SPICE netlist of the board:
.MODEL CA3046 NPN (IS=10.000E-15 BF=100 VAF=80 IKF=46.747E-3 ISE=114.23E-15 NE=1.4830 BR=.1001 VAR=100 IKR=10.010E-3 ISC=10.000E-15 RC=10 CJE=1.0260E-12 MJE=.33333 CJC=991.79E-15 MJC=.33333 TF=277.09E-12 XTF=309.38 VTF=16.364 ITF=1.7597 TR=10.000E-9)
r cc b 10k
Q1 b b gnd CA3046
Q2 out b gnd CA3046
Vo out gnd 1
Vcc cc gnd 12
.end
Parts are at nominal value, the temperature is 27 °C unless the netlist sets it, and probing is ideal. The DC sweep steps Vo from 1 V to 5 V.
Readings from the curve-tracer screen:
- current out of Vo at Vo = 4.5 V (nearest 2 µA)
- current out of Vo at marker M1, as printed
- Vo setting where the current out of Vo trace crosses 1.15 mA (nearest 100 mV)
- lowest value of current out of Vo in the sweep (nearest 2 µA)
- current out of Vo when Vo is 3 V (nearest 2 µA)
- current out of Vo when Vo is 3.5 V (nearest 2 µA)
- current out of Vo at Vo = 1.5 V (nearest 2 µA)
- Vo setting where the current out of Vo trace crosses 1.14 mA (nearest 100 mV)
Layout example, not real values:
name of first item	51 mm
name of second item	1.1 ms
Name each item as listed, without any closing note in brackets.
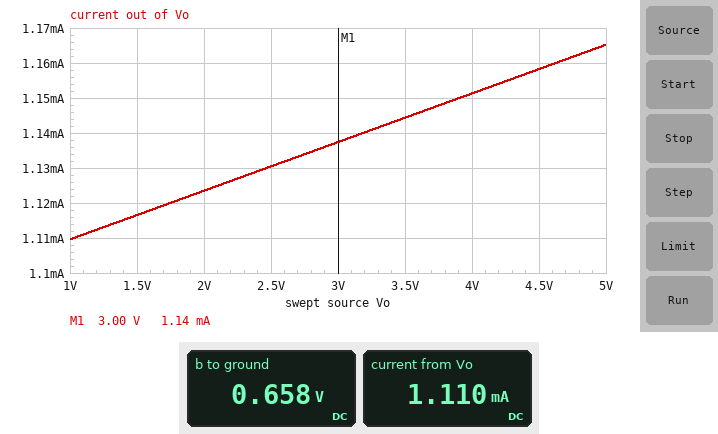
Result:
current out of Vo at Vo = 4.5 V	1.158 mA
current out of Vo at marker M1, as printed	1.14 mA
Vo setting where the current out of Vo trace crosses 1.15 mA	3.9 V
lowest value of current out of Vo in the sweep	1.110 mA
current out of Vo when Vo is 3 V	1.138 mA
current out of Vo when Vo is 3.5 V	1.144 mA
current out of Vo at Vo = 1.5 V	1.116 mA
Vo setting where the current out of Vo trace crosses 1.14 mA	3.2 V
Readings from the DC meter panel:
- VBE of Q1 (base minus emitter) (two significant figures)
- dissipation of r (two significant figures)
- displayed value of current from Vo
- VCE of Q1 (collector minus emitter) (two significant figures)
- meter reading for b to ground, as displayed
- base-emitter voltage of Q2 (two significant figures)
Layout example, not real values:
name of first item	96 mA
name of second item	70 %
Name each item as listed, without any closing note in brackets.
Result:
VBE of Q1 (base minus emitter)	660 mV
dissipation of r	13 mW
displayed value of current from Vo	1.110 mA
VCE of Q1 (collector minus emitter)	660 mV
meter reading for b to ground, as displayed	0.658 V
base-emitter voltage of Q2	660 mV
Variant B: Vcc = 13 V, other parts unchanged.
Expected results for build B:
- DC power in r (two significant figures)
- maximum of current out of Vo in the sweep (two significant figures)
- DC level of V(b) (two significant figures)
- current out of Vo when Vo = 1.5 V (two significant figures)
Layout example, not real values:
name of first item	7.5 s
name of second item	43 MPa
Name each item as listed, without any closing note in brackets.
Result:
DC power in r	15 mW
maximum of current out of Vo in the sweep	1.3 mA
DC level of V(b)	660 mV
current out of Vo when Vo = 1.5 V	1.2 mA
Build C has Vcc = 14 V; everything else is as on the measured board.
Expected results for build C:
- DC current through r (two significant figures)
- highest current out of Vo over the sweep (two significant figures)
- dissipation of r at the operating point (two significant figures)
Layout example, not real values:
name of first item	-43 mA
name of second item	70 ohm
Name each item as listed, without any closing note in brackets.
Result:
DC current through r	1.3 mA
highest current out of Vo over the sweep	1.4 mA
dissipation of r at the operating point	18 mW
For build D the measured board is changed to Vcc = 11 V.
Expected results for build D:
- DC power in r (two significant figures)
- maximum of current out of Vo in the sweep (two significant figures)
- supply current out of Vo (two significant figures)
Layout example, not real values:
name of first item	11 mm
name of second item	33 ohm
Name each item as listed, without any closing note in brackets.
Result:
DC power in r	11 mW
maximum of current out of Vo in the sweep	1.1 mA
supply current out of Vo	1.0 mA
